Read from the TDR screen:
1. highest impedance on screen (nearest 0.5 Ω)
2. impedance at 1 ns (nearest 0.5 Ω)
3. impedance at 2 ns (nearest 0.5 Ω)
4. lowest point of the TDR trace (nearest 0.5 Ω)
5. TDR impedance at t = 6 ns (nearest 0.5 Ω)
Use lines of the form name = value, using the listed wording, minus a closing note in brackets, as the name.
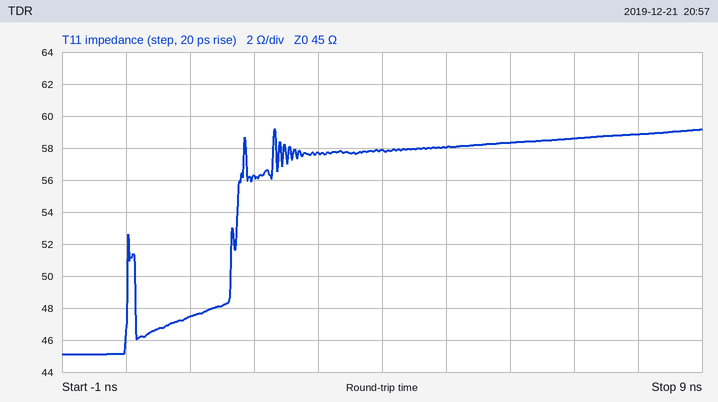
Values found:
highest impedance on screen = 59.0 Ω
impedance at 1 ns = 47.5 Ω
impedance at 2 ns = 56.5 Ω
lowest point of the TDR trace = 45.0 Ω
TDR impedance at t = 6 ns = 58.5 Ω
